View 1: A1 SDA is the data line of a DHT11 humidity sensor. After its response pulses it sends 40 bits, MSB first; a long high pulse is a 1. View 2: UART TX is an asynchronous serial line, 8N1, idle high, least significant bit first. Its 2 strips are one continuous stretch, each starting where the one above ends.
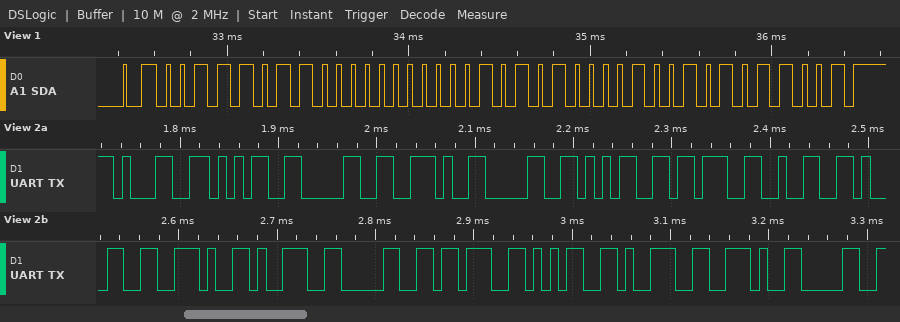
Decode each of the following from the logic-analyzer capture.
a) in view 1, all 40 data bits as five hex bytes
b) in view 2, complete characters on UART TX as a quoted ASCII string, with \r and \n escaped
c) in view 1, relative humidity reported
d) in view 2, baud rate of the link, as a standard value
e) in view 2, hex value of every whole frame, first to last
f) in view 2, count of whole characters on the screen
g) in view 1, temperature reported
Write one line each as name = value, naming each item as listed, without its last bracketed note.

in view 1, all 40 data bits as five hex bytes = 3B 00 15 09 59
in view 2, complete characters on UART TX as a quoted ASCII string, with \r and \n escaped = "150.05;21.90;59.0"
in view 1, relative humidity reported = 59 %
in view 2, baud rate of the link, as a standard value = 115200 baud
in view 2, hex value of every whole frame, first to last = 31 35 30 2E 30 35 3B 32 31 2E 39 30 3B 35 39 2E 30
in view 2, count of whole characters on the screen = 17
in view 1, temperature reported = 21.9 °C
